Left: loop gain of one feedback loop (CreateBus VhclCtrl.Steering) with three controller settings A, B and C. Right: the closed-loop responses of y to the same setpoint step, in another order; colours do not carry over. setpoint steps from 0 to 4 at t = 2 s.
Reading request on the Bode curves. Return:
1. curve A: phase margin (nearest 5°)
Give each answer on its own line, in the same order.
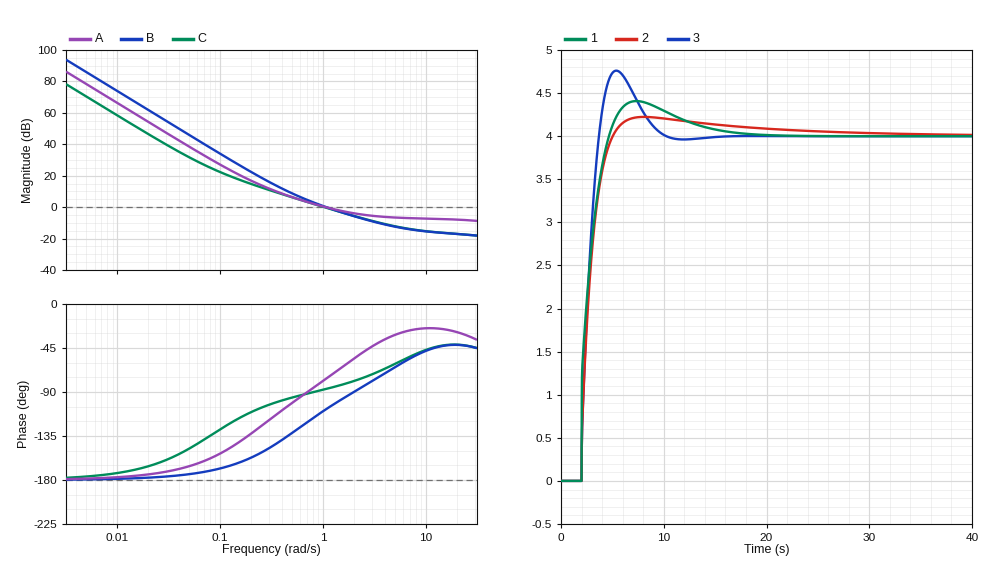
105°
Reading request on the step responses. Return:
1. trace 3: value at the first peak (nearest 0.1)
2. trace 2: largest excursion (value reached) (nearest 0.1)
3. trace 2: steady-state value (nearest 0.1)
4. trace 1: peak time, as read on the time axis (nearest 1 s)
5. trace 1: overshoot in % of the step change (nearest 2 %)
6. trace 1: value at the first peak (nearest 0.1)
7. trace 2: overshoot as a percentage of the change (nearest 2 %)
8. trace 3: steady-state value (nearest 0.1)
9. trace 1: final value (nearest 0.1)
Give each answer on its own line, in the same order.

4.8
4.2
4.0
7 s
10 %
4.4
6 %
4.0
4.0
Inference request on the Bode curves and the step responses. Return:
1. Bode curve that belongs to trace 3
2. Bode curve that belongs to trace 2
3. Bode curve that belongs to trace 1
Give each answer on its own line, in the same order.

B
C
A
